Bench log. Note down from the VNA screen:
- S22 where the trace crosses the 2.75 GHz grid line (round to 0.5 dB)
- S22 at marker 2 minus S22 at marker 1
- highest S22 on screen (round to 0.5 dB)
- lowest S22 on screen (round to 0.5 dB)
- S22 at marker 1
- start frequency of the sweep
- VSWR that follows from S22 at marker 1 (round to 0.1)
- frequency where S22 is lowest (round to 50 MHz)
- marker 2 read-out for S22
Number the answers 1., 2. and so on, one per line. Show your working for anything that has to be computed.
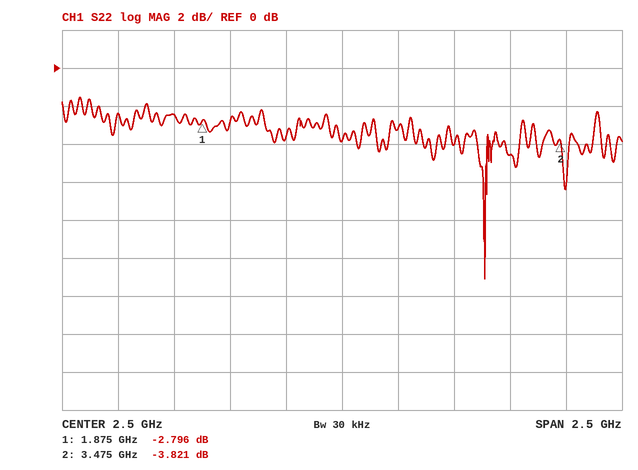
1. -3.0 dB
2. -3.821 − (-2.796) = -1.025 dB
3. -1.5 dB
4. -11.0 dB
5. -2.796 dB
6. 1.25 GHz
7. (1 + 0.7248)/(1 − 0.7248) ≈ 6.3
8. 3.15 GHz
9. -3.821 dB
